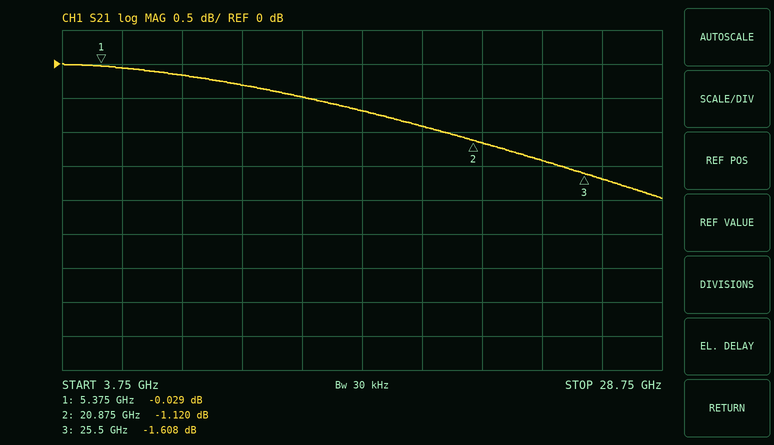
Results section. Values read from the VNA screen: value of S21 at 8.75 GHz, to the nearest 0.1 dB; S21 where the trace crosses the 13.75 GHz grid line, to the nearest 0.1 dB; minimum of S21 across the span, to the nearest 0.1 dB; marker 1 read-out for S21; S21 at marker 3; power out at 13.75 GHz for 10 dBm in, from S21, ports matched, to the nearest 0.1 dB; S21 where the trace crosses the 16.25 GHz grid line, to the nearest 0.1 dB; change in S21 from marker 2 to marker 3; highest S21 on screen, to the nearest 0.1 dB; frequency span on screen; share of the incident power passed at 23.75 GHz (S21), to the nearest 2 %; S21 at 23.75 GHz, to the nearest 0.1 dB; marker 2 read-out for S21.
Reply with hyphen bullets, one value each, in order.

- -0.2 dB
- -0.5 dB
- -2.0 dB
- -0.029 dB
- -1.608 dB
- 9.5 dBm
- -0.7 dB
- -0.488 dB
- 0.0 dB
- 25 GHz
- 72 %
- -1.4 dB
- -1.120 dB
